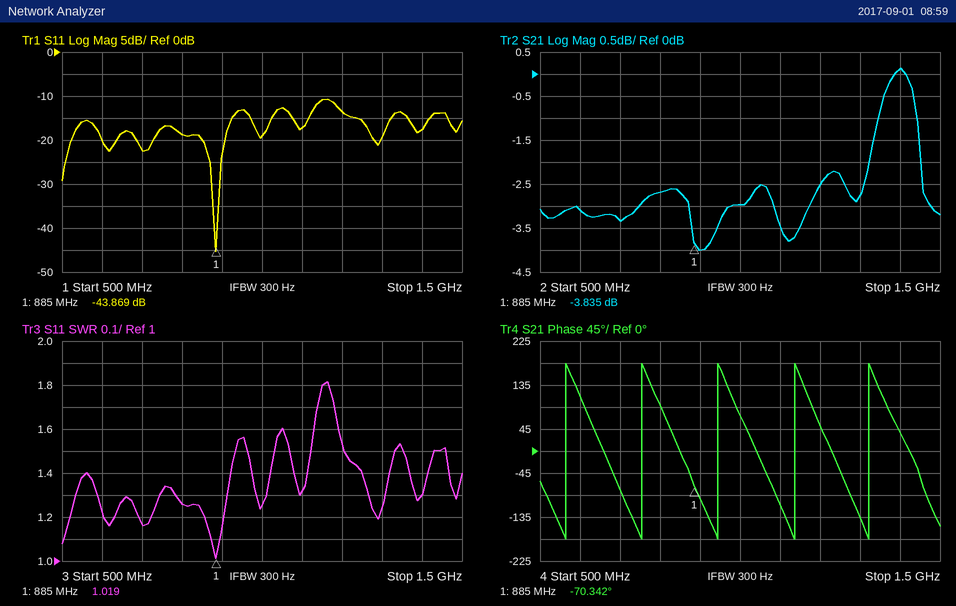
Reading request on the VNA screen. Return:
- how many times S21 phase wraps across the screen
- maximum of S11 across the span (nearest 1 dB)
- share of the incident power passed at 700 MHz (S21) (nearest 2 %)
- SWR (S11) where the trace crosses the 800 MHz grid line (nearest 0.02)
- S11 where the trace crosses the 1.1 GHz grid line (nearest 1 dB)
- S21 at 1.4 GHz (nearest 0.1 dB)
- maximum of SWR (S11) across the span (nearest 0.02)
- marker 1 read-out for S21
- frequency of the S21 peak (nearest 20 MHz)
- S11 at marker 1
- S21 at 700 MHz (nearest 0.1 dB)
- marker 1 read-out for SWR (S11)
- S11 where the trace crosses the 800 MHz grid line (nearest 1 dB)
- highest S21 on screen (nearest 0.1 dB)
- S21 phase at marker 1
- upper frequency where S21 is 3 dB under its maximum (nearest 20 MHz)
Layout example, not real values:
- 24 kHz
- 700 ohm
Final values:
- 5
- -11 dB
- 46 %
- 1.26
- -17 dB
- 0.1 dB
- 1.82
- -3.835 dB
- 1.40 GHz
- -43.869 dB
- -3.3 dB
- 1.019
- -19 dB
- 0.1 dB
- -70.342°
- 1.46 GHz
